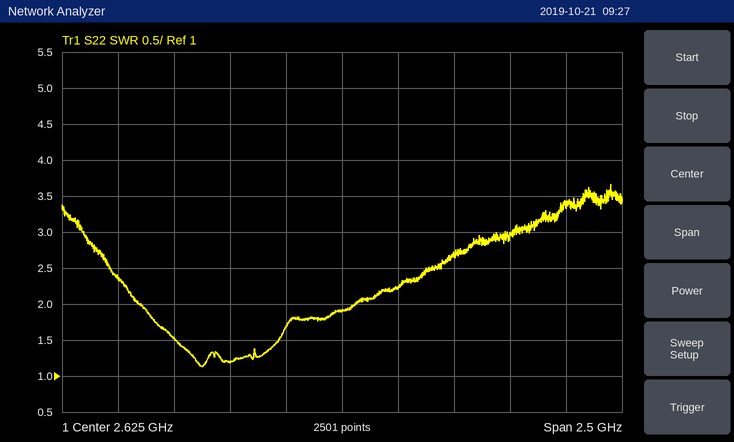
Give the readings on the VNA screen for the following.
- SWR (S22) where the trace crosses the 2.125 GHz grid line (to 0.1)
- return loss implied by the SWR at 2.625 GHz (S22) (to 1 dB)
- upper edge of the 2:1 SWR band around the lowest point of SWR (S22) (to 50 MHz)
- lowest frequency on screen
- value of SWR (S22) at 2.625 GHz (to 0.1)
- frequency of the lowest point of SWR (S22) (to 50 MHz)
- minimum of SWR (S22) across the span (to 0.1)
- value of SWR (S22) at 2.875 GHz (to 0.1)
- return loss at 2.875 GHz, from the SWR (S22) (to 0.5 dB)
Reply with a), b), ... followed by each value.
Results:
a) 1.2
b) 10 dB
c) 2.70 GHz
d) 1.375 GHz
e) 1.9
f) 2.00 GHz
g) 1.1
h) 2.2
i) 8.5 dB
